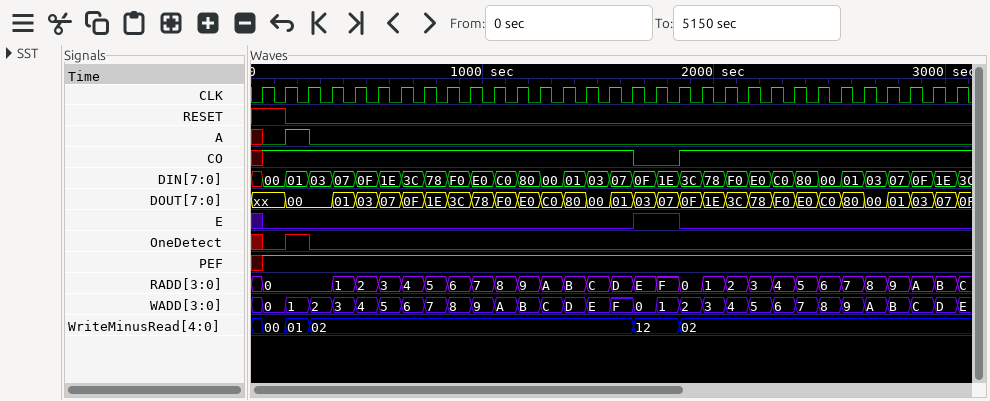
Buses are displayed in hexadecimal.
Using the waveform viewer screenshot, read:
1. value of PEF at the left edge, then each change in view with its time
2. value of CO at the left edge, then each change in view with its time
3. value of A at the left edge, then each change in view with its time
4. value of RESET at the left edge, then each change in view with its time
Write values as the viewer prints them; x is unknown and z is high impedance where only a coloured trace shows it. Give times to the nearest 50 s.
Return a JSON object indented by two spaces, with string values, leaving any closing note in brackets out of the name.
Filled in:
{
  "value of PEF at the left edge, then each change in view with its time": "x, 1 at 50 s",
  "value of CO at the left edge, then each change in view with its time": "x, 1 at 50 s, 0 at 1650 s, 1 at 1850 s",
  "value of A at the left edge, then each change in view with its time": "x, 0 at 50 s, 1 at 150 s, 0 at 250 s",
  "value of RESET at the left edge, then each change in view with its time": "1, 0 at 150 s"
}
